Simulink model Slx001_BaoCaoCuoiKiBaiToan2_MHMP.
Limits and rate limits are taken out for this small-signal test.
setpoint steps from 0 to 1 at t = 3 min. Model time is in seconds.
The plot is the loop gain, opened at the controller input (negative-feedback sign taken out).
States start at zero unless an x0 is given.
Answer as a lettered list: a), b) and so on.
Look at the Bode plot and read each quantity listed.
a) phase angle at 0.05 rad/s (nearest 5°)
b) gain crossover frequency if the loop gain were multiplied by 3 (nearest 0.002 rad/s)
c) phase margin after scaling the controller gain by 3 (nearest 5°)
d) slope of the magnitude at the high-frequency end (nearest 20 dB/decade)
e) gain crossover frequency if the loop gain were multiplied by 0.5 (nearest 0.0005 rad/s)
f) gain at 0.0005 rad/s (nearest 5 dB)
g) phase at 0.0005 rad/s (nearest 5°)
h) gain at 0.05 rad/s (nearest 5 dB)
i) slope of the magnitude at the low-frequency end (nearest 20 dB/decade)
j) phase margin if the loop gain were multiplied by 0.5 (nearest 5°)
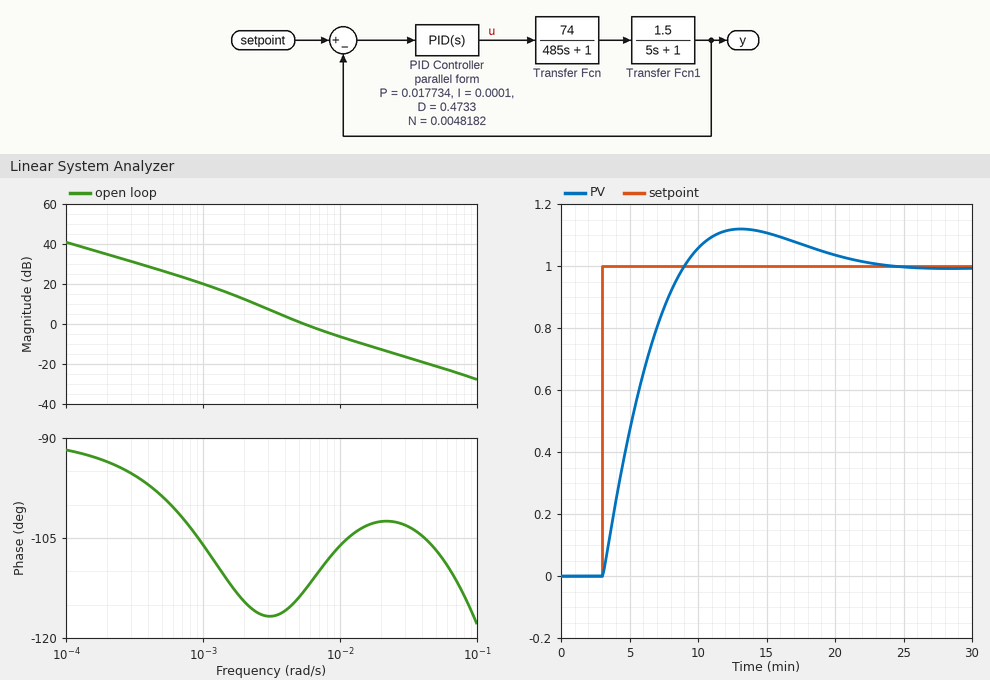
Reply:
a) -105°
b) 0.014 rad/s
c) 75°
d) -20 dB/decade
e) 0.0035 rad/s
f) 25 dB
g) -100°
h) -20 dB
i) -20 dB/decade
j) 65°
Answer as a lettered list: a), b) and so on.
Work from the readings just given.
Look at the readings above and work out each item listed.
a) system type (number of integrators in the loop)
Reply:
a) 1
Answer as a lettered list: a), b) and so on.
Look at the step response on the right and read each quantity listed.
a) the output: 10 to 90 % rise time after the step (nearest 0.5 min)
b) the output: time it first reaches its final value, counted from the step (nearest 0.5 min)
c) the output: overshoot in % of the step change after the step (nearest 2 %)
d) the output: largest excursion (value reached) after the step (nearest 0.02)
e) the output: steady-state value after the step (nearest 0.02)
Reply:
a) 4.5 min
b) 6.0 min
c) 12 %
d) 1.12
e) 1.00
